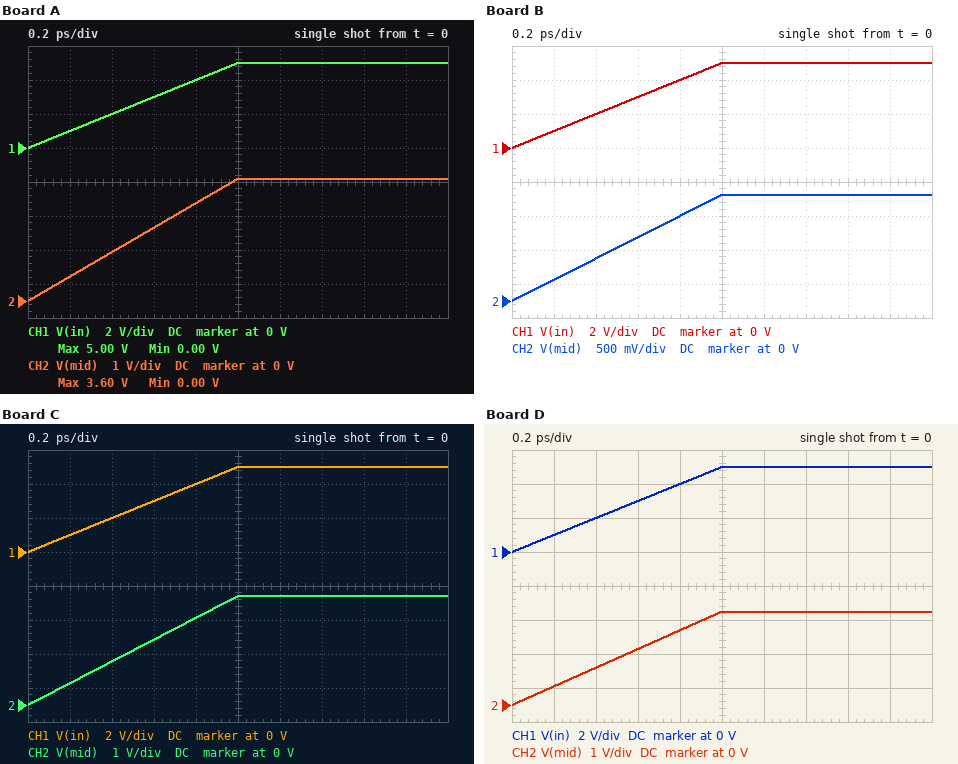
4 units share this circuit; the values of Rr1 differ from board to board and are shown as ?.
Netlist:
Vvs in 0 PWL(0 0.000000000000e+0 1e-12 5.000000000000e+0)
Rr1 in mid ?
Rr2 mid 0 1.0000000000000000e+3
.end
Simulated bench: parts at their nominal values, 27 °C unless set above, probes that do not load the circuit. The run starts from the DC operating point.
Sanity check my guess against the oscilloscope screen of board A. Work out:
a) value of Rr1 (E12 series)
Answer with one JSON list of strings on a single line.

["390 Ω"]
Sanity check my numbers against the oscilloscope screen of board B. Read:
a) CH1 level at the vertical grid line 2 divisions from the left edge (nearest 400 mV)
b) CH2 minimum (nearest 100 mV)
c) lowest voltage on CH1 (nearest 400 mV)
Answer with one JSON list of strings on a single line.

["2.0 V", "0 V", "0 V"]
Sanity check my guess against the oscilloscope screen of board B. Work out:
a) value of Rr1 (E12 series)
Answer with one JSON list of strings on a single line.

["2.2 kΩ"]
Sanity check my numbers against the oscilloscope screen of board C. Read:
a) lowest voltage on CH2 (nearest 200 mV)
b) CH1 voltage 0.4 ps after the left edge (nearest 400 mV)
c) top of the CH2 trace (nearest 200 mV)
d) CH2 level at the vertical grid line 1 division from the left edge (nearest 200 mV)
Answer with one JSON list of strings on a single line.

["0 V", "2.0 V", "3.2 V", "600 mV"]
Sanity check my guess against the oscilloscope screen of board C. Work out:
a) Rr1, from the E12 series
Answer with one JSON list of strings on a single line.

["560 Ω"]
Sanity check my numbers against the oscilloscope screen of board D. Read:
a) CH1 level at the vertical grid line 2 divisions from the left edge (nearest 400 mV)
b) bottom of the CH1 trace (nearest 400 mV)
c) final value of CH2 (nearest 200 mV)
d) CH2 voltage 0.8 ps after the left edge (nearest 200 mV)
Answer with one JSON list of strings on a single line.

["2.0 V", "0 V", "2.8 V", "2.2 V"]
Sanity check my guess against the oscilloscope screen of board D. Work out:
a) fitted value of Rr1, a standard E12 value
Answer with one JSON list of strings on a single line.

["820 Ω"]
